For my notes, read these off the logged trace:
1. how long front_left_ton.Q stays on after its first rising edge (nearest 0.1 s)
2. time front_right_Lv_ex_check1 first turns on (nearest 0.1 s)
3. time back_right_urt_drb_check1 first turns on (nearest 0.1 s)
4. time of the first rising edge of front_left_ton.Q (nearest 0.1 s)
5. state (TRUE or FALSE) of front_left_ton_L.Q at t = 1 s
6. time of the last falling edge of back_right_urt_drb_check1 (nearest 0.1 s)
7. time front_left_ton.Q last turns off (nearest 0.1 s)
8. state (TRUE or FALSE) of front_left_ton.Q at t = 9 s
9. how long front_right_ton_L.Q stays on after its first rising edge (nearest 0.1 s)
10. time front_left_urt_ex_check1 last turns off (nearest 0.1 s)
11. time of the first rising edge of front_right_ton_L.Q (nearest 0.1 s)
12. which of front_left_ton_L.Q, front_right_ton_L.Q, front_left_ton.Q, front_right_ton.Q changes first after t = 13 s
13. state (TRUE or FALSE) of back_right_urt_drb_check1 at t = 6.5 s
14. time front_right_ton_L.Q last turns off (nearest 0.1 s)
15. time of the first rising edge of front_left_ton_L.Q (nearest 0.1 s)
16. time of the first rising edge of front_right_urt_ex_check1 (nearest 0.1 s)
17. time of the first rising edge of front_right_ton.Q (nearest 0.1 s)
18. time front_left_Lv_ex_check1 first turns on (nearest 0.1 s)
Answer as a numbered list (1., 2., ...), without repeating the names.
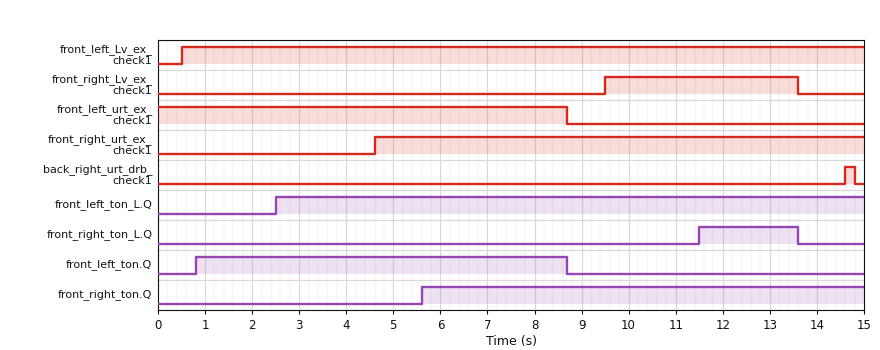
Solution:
1. 7.9 s
2. 9.5 s
3. 14.6 s
4. 0.8 s
5. FALSE
6. 14.8 s
7. 8.7 s
8. FALSE
9. 2.1 s
10. 8.7 s
11. 11.5 s
12. front_right_ton_L.Q
13. FALSE
14. 13.6 s
15. 2.5 s
16. 4.6 s
17. 5.6 s
18. 0.5 s
